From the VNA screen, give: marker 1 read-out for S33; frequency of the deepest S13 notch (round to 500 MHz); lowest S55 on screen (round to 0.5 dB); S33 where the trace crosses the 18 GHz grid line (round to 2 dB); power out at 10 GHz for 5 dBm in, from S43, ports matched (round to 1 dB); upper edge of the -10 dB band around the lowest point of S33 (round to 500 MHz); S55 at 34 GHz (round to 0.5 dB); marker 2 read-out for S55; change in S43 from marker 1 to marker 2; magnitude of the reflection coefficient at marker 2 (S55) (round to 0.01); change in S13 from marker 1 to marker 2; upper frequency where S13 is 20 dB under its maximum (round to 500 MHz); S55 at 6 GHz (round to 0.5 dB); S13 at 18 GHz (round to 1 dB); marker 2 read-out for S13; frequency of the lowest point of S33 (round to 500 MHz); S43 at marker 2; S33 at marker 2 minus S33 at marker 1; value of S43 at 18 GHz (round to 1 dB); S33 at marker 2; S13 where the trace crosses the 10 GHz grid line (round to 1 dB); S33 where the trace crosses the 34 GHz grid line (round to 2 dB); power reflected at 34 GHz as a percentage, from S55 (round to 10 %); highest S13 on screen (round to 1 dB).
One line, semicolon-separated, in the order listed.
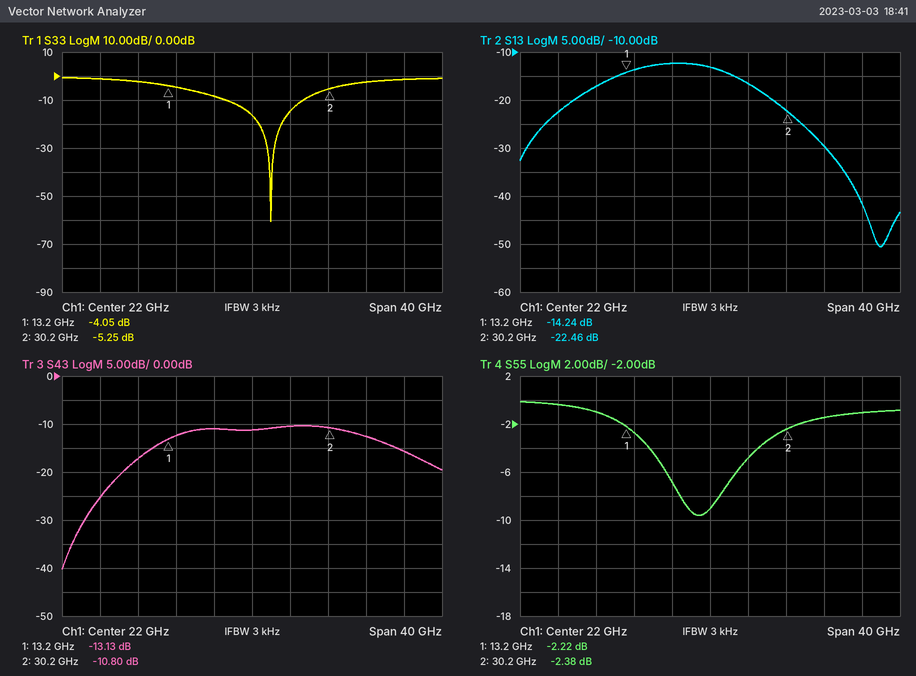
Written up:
-4.05 dB; 40.0 GHz; -9.5 dB; -8 dB; -12 dBm; 27.5 GHz; -1.5 dB; -2.38 dB; 2.33 dB; 0.76; -8.22 dB; 35.0 GHz; -0.5 dB; -12 dB; -22.46 dB; 24.0 GHz; -10.80 dB; -1.20 dB; -11 dB; -5.25 dB; -17 dB; -2 dB; 70 %; -12 dB
